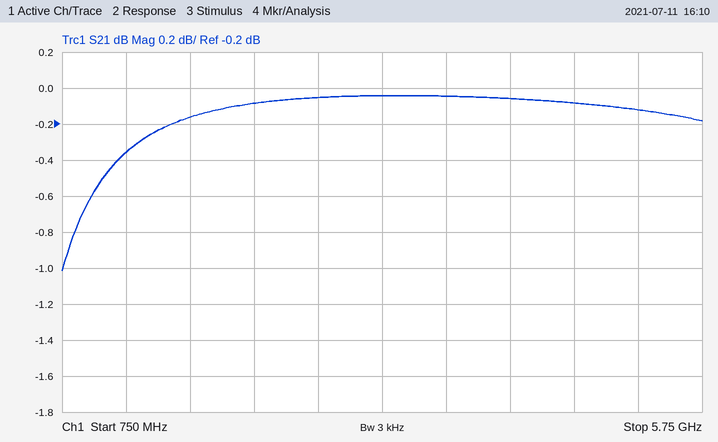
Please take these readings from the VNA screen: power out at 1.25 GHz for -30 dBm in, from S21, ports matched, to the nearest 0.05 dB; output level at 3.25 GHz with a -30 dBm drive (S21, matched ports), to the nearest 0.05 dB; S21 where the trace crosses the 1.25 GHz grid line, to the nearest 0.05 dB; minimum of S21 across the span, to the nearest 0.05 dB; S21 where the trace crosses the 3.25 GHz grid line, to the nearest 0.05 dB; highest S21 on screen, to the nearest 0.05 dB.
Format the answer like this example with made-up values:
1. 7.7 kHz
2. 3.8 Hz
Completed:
1. -30.35 dBm
2. -30.05 dBm
3. -0.35 dB
4. -1.00 dB
5. -0.05 dB
6. -0.05 dB
